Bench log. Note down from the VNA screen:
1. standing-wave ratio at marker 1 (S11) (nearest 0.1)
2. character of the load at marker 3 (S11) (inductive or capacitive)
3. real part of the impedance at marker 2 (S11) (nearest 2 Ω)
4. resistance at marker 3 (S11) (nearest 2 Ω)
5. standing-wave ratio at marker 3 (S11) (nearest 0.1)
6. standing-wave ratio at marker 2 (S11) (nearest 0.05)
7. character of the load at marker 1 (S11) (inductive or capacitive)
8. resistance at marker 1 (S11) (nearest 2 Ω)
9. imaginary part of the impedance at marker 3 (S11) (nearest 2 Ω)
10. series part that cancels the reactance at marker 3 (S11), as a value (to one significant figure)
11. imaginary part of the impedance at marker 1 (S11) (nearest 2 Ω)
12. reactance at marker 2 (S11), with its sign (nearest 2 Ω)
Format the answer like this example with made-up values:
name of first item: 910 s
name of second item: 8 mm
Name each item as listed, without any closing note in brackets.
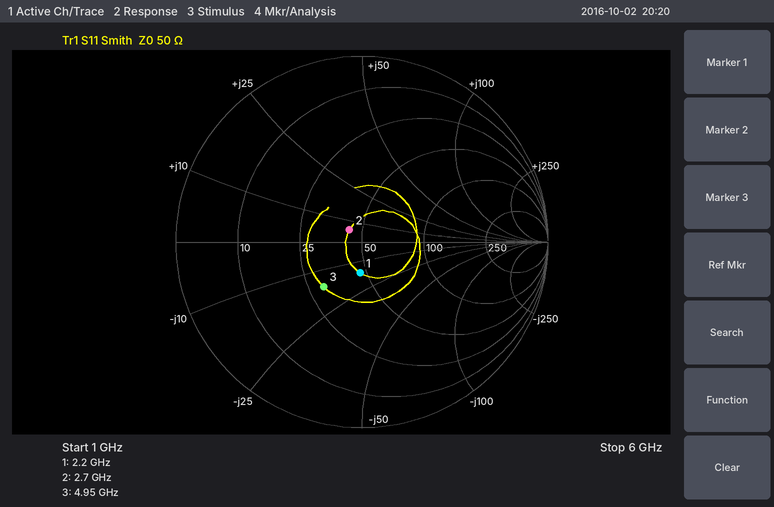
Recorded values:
standing-wave ratio at marker 1 (S11): 1.4
character of the load at marker 3 (S11): capacitive
real part of the impedance at marker 2 (S11): 44 Ω
resistance at marker 3 (S11): 30 Ω
standing-wave ratio at marker 3 (S11): 1.9
standing-wave ratio at marker 2 (S11): 1.20
character of the load at marker 1 (S11): capacitive
resistance at marker 1 (S11): 46 Ω
imaginary part of the impedance at marker 3 (S11): -16 Ω
series part that cancels the reactance at marker 3 (S11), as a value: 500 pH
imaginary part of the impedance at marker 1 (S11): -16 Ω
reactance at marker 2 (S11), with its sign: +6 Ω
